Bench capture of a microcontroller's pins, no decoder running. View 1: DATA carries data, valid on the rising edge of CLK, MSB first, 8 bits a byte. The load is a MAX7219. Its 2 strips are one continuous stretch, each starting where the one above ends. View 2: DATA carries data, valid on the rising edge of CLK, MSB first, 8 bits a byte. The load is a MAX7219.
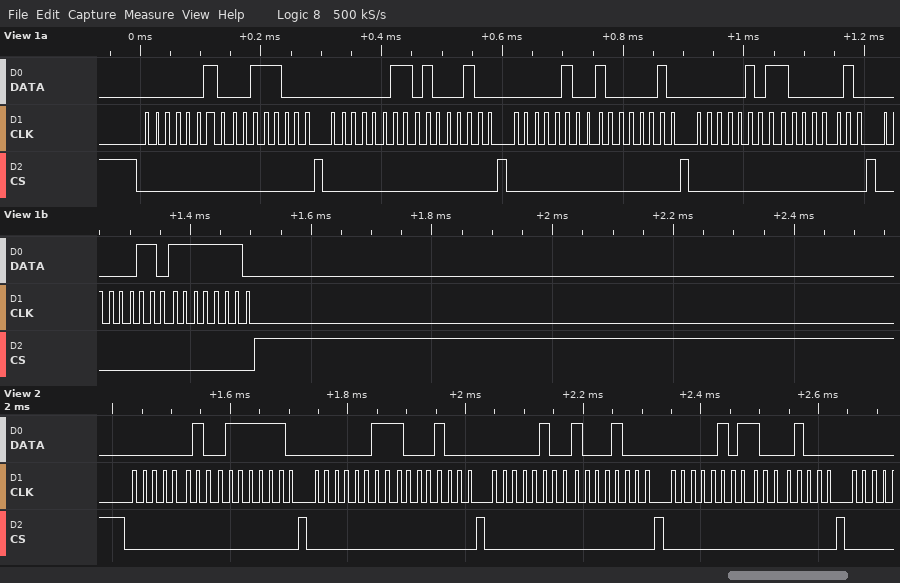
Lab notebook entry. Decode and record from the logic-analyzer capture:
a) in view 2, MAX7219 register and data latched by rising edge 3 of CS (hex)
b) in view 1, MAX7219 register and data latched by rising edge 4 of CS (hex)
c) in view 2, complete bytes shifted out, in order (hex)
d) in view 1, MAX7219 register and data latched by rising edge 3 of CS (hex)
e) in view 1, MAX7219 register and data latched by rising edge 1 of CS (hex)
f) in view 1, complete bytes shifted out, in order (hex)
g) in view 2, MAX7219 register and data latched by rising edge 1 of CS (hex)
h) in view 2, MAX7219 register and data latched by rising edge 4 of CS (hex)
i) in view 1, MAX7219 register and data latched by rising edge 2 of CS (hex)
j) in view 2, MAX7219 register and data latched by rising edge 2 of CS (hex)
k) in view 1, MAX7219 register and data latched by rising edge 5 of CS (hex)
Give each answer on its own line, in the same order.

register 0x4, data 0x88
register 0x5, data 0x82
02 7E 03 88 04 88 05 88
register 0x4, data 0x82
register 0x2, data 0x38
02 38 03 44 04 82 05 82 06 FE
register 0x2, data 0x7E
register 0x5, data 0x88
register 0x3, data 0x44
register 0x3, data 0x88
register 0x6, data 0xFE
